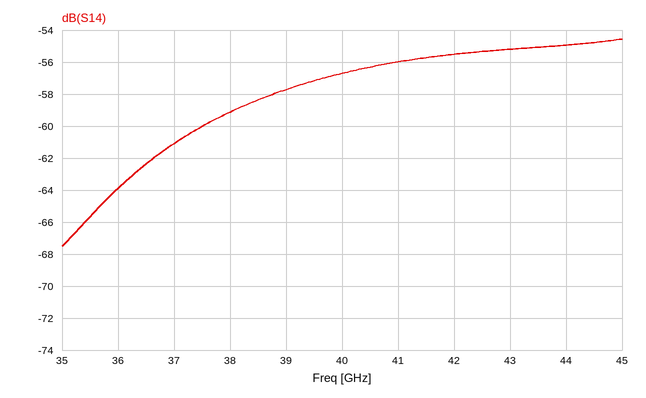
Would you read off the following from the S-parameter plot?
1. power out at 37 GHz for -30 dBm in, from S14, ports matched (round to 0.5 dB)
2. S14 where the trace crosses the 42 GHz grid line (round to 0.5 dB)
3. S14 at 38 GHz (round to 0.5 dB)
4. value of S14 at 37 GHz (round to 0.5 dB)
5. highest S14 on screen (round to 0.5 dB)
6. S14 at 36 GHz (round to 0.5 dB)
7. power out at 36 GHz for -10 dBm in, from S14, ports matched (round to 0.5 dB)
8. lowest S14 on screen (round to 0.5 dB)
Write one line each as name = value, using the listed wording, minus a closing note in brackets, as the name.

power out at 37 GHz for -30 dBm in, from S14, ports matched = -91.0 dBm
S14 where the trace crosses the 42 GHz grid line = -55.5 dB
S14 at 38 GHz = -59.0 dB
value of S14 at 37 GHz = -61.0 dB
highest S14 on screen = -54.5 dB
S14 at 36 GHz = -64.0 dB
power out at 36 GHz for -10 dBm in, from S14, ports matched = -74.0 dBm
lowest S14 on screen = -67.5 dB
